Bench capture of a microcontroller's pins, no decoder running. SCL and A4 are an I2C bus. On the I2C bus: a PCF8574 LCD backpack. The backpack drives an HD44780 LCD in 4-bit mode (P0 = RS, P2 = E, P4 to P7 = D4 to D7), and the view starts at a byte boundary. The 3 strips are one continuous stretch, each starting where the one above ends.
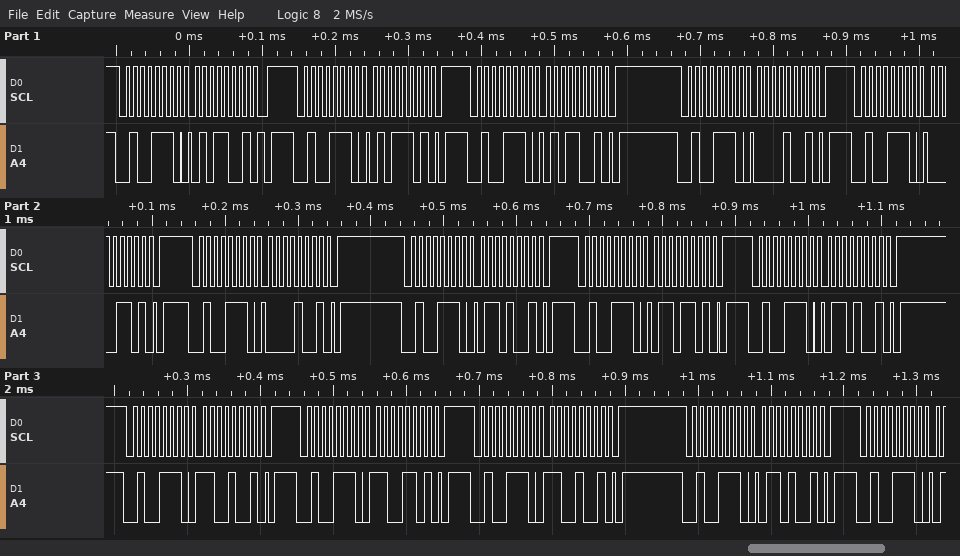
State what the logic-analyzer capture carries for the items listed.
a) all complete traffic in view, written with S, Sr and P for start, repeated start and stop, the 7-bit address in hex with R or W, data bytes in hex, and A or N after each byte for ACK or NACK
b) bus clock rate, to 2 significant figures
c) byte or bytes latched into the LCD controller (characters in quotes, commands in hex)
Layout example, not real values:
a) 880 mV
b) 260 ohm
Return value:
a) S 27W A 59 A P S 27W A 5D A P S 27W A 59 A P S 27W A 09 A P S 27W A 0D A P S 27W A 09 A P S 27W A 69 A P S 27W A 6D A P S 27W A 69 A P S 27W A C9 A P S 27W A CD A P S 27W A C9 A P S 27W A 69 A P S 27W A
b) 100 kHz
c) 'P' 'l'
